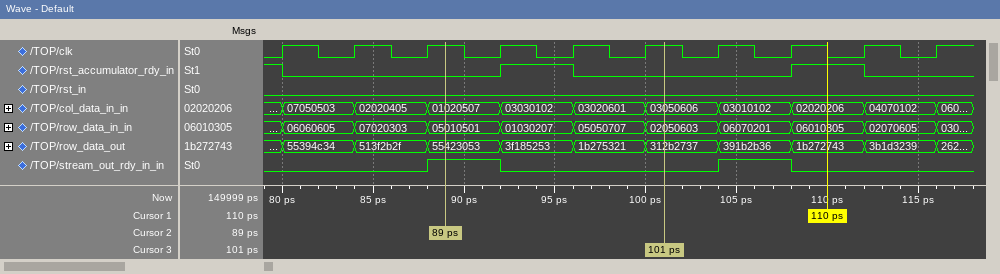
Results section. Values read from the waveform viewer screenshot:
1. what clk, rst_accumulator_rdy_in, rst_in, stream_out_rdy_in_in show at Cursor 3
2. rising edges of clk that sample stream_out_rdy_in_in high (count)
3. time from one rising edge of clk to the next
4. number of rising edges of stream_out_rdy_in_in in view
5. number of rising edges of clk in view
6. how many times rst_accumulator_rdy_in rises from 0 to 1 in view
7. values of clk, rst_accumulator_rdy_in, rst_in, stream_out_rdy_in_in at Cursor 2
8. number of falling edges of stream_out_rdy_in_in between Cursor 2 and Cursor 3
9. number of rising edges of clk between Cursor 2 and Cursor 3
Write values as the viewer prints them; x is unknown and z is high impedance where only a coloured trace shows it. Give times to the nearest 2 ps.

clk=1, rst_accumulator_rdy_in=0, rst_in=0, stream_out_rdy_in_in=0
2
4 ps
2
10
2
clk=1, rst_accumulator_rdy_in=0, rst_in=0, stream_out_rdy_in_in=1
1
3
